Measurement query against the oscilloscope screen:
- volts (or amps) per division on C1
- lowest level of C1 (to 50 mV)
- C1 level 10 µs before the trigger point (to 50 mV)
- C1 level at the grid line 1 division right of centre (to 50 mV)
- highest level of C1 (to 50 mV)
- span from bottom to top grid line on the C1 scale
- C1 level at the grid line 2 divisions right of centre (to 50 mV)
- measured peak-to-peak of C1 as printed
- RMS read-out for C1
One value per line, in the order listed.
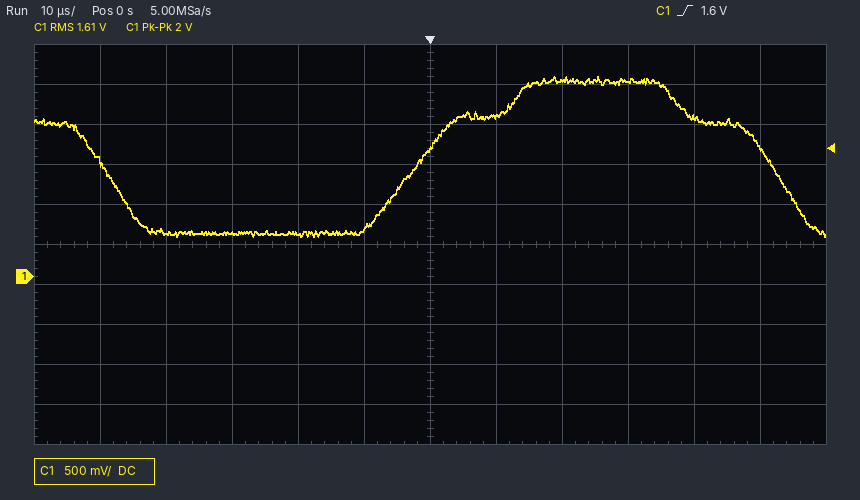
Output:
500 mV
500 mV
600 mV
2.00 V
2.50 V
5 V
2.45 V
2 V
1.61 V
